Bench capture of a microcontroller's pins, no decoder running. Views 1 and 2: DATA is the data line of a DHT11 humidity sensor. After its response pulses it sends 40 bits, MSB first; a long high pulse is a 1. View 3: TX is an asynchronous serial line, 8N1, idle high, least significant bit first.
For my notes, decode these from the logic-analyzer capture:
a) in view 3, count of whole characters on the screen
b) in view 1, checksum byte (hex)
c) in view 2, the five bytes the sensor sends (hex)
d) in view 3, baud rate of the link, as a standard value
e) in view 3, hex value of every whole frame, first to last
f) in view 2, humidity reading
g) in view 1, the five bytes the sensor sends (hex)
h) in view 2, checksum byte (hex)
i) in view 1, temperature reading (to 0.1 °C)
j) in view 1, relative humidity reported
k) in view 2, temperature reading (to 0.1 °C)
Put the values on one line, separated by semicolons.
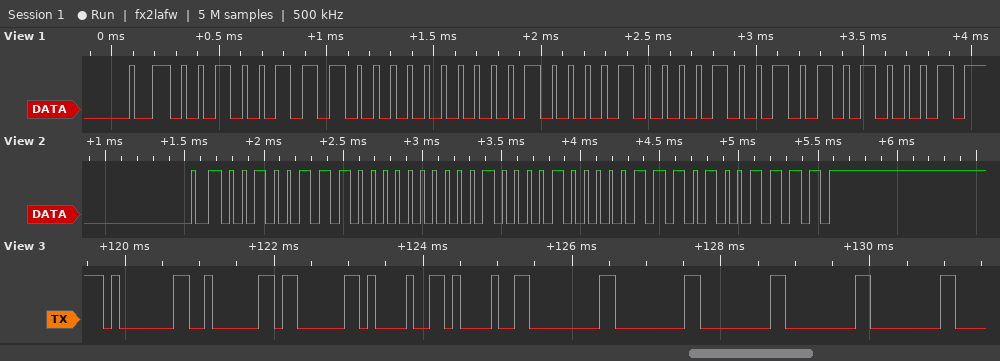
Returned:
10; 0x51; 27 00 21 07 4F; 9600 baud; 01 02 03 21 21 00 00 00 00 00; 39 %; 27 00 21 09 51; 0x4F; 33.9 °C; 39 %; 33.7 °C
